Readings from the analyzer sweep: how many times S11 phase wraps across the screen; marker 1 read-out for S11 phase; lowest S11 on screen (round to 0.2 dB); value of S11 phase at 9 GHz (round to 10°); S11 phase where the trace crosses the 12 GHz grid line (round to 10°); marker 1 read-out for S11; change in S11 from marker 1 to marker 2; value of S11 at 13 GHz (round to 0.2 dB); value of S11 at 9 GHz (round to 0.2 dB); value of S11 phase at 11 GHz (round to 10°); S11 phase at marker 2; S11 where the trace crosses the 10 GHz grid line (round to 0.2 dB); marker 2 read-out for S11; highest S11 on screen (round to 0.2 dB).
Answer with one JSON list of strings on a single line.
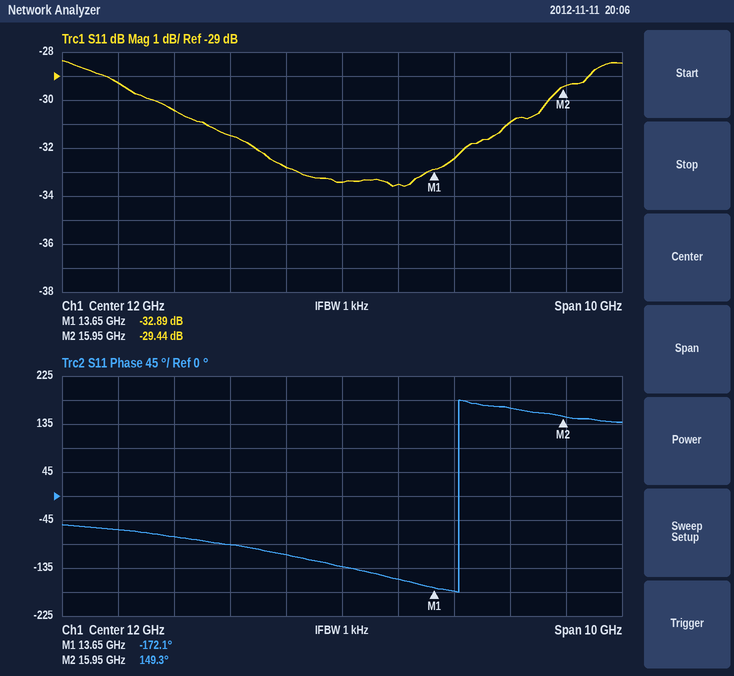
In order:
["1", "-172.1°", "-33.6 dB", "-80°", "-130°", "-32.89 dB", "3.45 dB", "-33.6 dB", "-30.4 dB", "-110°", "149.3°", "-31.4 dB", "-29.44 dB", "-28.4 dB"]
